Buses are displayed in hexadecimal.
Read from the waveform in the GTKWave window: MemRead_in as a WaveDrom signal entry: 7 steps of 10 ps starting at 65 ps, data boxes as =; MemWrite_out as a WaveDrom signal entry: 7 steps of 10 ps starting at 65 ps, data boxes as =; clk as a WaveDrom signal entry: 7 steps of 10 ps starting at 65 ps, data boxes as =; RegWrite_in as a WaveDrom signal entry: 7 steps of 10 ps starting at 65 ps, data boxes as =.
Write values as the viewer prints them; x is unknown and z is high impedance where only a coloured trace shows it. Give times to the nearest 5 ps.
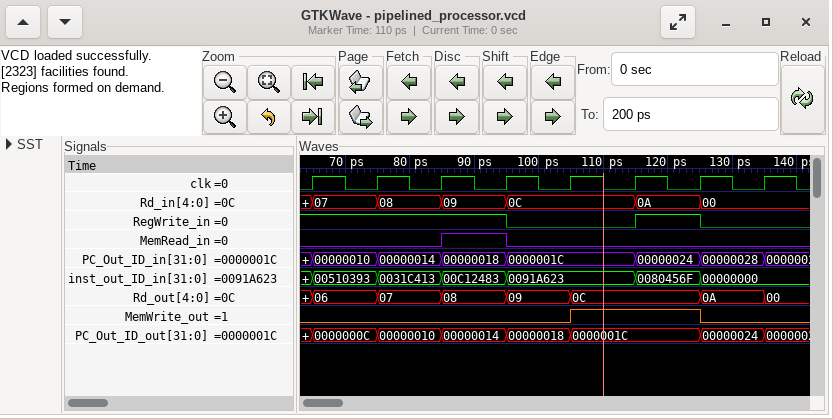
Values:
{name: 'MemRead_in', wave: '0.10...'}
{name: 'MemWrite_out', wave: '0...1.0'}
{name: 'clk', wave: 'p......'}
{name: 'RegWrite_in', wave: '1..0.10'}
